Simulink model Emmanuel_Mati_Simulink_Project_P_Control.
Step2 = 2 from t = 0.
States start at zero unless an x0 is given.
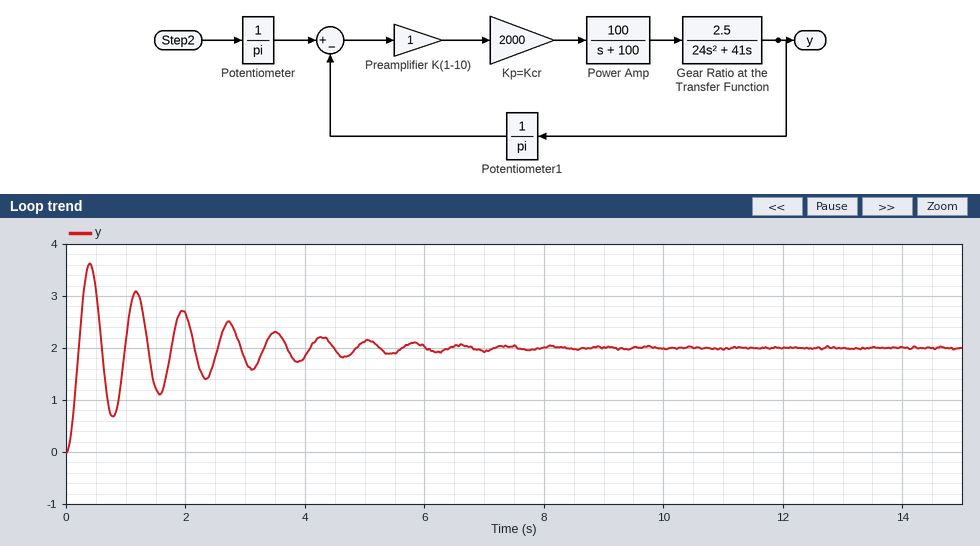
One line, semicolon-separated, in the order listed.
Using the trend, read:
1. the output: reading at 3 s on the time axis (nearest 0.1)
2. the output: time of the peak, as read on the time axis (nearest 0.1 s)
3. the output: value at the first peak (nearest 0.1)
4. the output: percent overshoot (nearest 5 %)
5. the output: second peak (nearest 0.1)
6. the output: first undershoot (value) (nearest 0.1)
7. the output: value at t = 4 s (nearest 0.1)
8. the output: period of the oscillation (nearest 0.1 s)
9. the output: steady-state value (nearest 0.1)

1.8; 0.4 s; 3.6; 80 %; 3.1; 0.7; 1.8; 0.8 s; 2.0
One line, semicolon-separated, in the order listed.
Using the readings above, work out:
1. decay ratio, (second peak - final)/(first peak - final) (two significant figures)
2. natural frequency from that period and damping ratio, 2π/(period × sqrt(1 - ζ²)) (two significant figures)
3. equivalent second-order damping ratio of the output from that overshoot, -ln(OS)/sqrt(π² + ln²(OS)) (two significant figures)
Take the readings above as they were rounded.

0.69; 7.9 rad/s; 0.071
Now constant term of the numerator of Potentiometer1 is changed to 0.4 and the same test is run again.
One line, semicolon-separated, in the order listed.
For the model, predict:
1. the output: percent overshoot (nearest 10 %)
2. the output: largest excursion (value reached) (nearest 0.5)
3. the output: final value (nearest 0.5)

60 %; 8.0; 5.0
